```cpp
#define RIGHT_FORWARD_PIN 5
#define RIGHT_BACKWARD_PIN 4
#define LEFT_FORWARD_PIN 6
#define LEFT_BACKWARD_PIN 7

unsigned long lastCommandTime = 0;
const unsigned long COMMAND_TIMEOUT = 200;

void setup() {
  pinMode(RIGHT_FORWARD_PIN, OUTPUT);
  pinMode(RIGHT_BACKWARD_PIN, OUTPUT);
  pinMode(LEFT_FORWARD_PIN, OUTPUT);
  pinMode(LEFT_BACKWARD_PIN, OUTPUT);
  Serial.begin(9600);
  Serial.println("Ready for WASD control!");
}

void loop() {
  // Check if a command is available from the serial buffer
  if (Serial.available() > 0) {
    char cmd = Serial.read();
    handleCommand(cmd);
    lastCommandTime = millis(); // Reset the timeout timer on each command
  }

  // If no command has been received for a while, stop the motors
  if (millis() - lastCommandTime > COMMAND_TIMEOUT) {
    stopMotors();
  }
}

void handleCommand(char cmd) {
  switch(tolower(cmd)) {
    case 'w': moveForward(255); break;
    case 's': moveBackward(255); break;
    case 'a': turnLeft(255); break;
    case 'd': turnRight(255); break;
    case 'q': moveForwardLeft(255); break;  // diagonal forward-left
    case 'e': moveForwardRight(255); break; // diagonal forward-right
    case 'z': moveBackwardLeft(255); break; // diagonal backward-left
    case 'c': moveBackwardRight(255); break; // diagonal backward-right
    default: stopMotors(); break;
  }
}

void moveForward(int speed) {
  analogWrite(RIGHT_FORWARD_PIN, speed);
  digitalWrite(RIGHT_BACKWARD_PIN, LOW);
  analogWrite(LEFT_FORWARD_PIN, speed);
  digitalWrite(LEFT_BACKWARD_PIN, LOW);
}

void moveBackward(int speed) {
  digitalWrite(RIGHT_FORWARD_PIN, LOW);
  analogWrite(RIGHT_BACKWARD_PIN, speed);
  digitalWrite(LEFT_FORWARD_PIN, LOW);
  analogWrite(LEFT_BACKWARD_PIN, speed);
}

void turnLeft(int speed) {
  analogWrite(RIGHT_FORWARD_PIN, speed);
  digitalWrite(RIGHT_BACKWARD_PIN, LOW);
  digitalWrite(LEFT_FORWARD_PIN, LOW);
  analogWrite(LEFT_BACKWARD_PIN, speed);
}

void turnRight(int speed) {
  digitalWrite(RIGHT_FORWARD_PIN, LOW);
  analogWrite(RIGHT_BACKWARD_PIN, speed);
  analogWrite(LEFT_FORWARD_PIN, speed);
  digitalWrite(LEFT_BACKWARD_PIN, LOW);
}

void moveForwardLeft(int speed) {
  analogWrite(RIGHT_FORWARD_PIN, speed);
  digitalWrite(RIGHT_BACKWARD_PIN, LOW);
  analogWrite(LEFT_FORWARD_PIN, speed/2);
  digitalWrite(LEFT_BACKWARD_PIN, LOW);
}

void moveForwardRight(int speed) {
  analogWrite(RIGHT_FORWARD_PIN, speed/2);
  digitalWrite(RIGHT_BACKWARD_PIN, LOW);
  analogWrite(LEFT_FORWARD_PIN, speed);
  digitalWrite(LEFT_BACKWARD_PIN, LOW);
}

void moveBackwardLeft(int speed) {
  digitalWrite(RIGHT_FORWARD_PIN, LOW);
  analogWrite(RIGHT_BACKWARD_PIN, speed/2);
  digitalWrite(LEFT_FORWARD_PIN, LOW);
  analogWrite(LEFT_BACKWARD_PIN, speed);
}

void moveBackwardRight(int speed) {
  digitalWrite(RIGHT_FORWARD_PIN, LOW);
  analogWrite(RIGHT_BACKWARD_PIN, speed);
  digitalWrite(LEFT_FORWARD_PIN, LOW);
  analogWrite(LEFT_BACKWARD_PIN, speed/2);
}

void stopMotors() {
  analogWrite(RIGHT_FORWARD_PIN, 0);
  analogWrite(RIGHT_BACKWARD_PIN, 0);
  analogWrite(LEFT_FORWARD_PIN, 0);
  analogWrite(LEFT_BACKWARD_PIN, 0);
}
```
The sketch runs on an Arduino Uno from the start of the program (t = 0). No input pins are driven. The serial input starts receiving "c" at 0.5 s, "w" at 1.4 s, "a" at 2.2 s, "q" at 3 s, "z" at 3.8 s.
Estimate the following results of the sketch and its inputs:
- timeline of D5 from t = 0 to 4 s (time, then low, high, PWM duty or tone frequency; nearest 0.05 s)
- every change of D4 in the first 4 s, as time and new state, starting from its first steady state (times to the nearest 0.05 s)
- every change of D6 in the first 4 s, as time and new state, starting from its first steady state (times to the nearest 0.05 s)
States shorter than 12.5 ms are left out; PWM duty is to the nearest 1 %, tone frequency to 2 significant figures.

0 s low; 1.4 s high; 1.6 s low; 2.2 s high; 2.4 s low; 3 s high; 3.2 s low
0 s low; 0.5 s high; 0.7 s low
0 s low; 1.4 s high; 1.6 s low; 3 s PWM 50 %; 3.2 s low
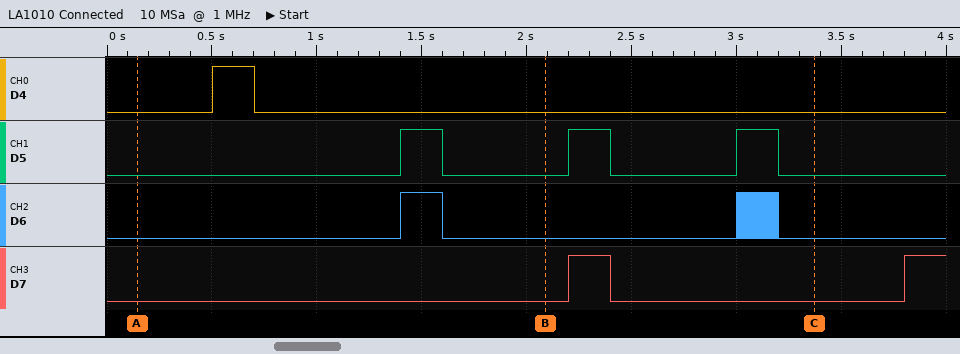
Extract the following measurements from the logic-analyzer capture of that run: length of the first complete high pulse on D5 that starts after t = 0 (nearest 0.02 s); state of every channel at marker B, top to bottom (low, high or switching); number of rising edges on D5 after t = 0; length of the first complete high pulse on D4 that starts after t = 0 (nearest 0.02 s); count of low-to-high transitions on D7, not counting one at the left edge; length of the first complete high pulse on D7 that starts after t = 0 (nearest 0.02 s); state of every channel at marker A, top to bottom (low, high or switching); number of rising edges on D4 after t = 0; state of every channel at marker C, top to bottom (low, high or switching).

0.20 s
D4 low, D5 low, D6 low, D7 low
3
0.20 s
2
0.20 s
D4 low, D5 low, D6 low, D7 low
1
D4 low, D5 low, D6 low, D7 low
